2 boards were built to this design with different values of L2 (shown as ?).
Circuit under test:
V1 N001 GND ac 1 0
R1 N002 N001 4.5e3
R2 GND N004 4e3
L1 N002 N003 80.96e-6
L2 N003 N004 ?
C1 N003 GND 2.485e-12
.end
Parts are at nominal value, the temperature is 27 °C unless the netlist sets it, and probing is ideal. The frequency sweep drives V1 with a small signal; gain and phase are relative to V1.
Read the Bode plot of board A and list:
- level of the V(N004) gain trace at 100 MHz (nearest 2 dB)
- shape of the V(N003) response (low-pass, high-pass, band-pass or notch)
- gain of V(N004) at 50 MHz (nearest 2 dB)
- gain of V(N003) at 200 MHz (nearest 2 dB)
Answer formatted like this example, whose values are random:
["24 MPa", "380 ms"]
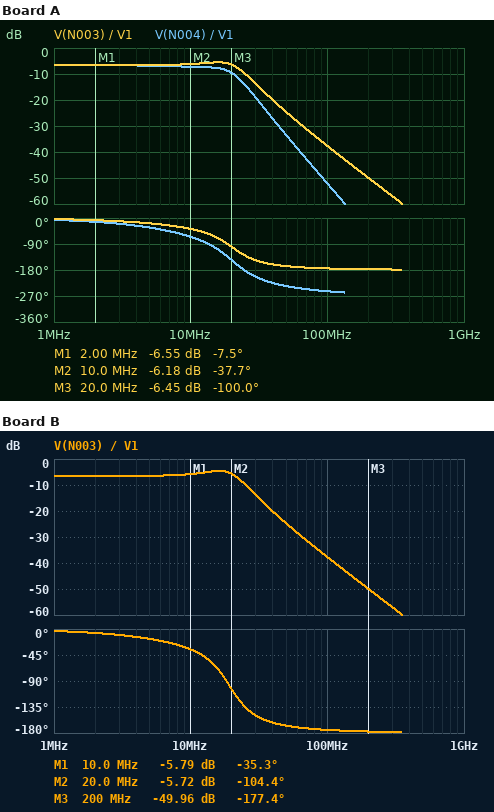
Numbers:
["-52 dB", "low-pass", "-34 dB", "-50 dB"]
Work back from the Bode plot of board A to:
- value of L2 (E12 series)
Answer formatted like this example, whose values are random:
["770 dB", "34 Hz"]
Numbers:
["33 µH"]
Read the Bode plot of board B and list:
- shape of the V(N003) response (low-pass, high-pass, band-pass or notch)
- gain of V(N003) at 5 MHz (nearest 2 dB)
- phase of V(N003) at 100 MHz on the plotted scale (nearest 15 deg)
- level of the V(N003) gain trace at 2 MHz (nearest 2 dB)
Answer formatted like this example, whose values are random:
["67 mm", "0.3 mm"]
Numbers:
["low-pass", "-6 dB", "-180 deg", "-6 dB"]
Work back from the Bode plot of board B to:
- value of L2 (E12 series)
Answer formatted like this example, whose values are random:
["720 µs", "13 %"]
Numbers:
["39 µH"]
